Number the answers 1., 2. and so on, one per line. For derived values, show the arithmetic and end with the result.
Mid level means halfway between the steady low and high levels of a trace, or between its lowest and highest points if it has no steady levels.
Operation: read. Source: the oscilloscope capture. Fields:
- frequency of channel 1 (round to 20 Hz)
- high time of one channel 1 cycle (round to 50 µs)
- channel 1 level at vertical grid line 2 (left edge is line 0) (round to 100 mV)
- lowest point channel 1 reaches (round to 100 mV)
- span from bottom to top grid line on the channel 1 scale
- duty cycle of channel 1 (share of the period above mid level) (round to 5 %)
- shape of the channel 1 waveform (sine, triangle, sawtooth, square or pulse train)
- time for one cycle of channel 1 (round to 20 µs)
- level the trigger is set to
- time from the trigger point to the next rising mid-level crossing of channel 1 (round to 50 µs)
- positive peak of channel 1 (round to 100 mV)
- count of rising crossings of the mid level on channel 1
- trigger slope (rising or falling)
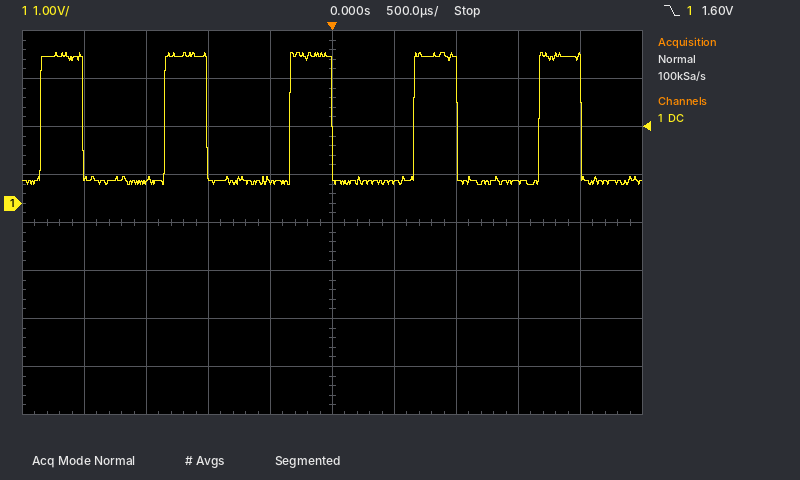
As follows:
1. 1 / 1.00 ms ≈ 1.00 kHz
2. 350 µs
3. 500 mV
4. 400 mV
5. 8 V
6. 350 µs / 1.00 ms ≈ 35 %
7. pulse train
8. 1.00 ms
9. 1.60 V
10. 650 µs
11. 3.1 V
12. 5
13. falling
